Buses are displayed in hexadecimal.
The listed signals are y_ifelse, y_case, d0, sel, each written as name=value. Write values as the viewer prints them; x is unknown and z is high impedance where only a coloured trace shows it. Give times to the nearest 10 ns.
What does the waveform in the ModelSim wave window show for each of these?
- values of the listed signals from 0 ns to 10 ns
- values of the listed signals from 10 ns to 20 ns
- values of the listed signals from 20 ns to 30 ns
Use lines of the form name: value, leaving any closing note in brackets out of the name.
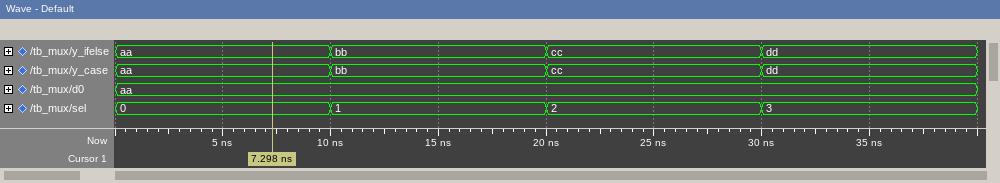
values of the listed signals from 0 ns to 10 ns: y_ifelse=aa, y_case=aa, d0=aa, sel=0
values of the listed signals from 10 ns to 20 ns: y_ifelse=bb, y_case=bb, d0=aa, sel=1
values of the listed signals from 20 ns to 30 ns: y_ifelse=cc, y_case=cc, d0=aa, sel=2
